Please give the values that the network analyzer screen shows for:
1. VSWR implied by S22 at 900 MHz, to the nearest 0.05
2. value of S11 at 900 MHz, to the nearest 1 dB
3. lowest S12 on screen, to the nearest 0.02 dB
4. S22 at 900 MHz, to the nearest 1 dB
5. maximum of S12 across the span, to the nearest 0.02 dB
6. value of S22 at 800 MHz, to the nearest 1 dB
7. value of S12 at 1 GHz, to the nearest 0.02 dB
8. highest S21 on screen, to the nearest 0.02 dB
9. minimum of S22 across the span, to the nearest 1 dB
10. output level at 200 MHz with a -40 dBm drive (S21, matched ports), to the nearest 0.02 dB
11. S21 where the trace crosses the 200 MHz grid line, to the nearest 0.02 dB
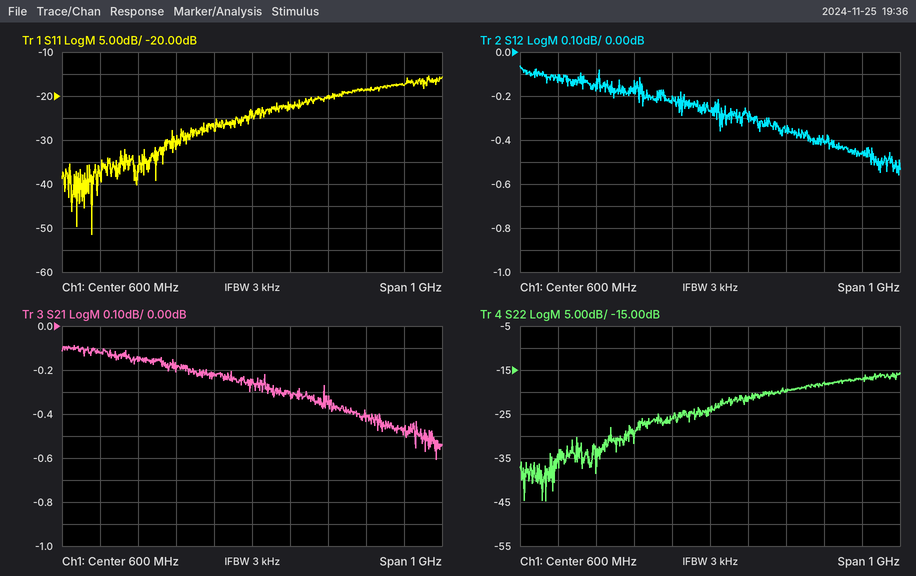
1.30
-19 dB
-0.56 dB
-18 dB
-0.06 dB
-20 dB
-0.46 dB
-0.08 dB
-45 dB
-40.12 dBm
-0.12 dB
